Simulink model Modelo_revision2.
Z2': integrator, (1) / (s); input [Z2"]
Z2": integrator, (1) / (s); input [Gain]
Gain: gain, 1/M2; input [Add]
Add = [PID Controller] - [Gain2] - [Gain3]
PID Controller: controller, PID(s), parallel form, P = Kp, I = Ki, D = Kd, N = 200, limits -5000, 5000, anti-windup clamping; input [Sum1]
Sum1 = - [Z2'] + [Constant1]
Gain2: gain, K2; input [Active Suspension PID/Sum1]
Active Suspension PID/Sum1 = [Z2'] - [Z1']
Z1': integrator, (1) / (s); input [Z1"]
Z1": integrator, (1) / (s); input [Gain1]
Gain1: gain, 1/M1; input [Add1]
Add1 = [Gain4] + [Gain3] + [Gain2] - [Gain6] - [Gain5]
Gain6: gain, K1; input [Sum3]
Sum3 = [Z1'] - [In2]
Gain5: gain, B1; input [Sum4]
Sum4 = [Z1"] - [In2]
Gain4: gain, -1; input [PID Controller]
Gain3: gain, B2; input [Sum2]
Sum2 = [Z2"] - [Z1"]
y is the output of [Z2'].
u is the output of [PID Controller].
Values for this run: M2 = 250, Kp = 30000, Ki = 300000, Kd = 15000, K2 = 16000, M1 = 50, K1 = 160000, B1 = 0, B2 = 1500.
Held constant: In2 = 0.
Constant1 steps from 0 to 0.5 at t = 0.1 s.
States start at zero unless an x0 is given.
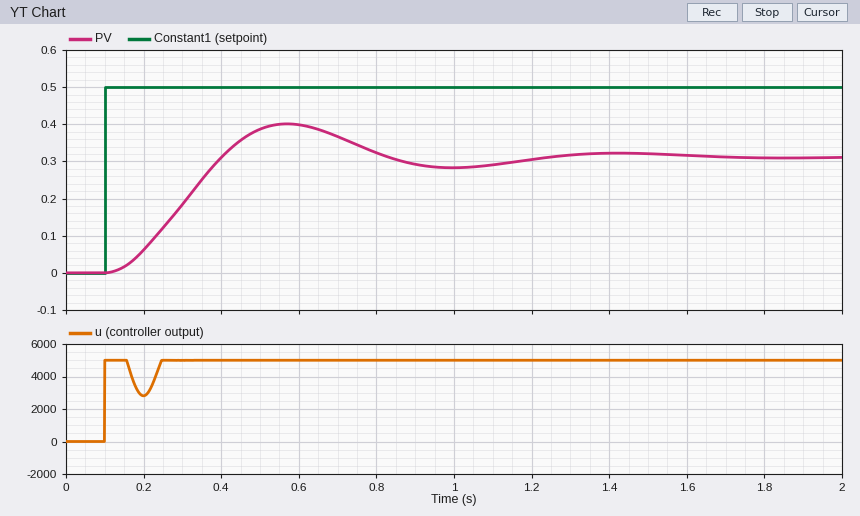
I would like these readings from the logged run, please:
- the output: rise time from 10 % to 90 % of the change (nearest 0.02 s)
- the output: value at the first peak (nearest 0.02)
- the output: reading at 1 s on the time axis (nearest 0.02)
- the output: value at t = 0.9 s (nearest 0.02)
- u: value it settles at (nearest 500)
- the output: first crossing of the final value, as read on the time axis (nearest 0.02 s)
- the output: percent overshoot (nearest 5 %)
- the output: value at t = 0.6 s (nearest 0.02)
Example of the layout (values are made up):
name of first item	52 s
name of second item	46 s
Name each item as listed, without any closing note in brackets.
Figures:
the output: rise time from 10 % to 90 % of the change	0.20 s
the output: value at the first peak	0.40
the output: reading at 1 s on the time axis	0.28
the output: value at t = 0.9 s	0.30
u: value it settles at	5000
the output: first crossing of the final value, as read on the time axis	0.40 s
the output: percent overshoot	30 %
the output: value at t = 0.6 s	0.40
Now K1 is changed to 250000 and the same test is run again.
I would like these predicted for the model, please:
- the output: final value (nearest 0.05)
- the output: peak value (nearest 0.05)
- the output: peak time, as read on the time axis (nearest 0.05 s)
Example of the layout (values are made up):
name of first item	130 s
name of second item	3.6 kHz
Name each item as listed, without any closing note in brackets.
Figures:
the output: final value	0.30
the output: peak value	0.40
the output: peak time, as read on the time axis	0.55 s
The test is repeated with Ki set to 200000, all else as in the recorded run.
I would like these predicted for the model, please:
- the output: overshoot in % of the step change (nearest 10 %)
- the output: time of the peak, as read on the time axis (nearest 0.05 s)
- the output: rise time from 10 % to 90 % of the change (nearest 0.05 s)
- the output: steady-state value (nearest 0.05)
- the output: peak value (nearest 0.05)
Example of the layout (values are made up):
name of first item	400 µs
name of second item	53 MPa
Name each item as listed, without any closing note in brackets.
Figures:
the output: overshoot in % of the step change	20 %
the output: time of the peak, as read on the time axis	0.60 s
the output: rise time from 10 % to 90 % of the change	0.25 s
the output: steady-state value	0.30
the output: peak value	0.40
